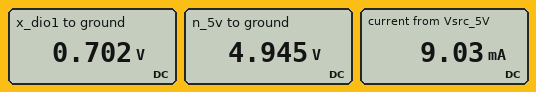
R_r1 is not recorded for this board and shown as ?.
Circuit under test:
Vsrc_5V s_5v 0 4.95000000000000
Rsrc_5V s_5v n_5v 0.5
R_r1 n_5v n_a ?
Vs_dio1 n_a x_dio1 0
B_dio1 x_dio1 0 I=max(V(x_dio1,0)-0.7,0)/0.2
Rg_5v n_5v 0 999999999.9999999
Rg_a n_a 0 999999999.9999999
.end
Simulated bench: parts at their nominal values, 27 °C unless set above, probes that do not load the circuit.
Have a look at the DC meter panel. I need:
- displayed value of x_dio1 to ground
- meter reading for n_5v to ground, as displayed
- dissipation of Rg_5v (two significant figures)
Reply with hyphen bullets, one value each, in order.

- 0.702 V
- 4.945 V
- 24 nW
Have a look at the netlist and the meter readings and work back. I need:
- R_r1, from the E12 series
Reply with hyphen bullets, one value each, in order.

- 470 Ω
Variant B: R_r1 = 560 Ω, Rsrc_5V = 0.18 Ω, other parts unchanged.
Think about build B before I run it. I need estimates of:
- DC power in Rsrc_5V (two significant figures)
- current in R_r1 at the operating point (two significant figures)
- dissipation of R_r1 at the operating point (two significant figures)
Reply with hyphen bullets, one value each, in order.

- 10 µW
- 7.6 mA
- 32 mW
